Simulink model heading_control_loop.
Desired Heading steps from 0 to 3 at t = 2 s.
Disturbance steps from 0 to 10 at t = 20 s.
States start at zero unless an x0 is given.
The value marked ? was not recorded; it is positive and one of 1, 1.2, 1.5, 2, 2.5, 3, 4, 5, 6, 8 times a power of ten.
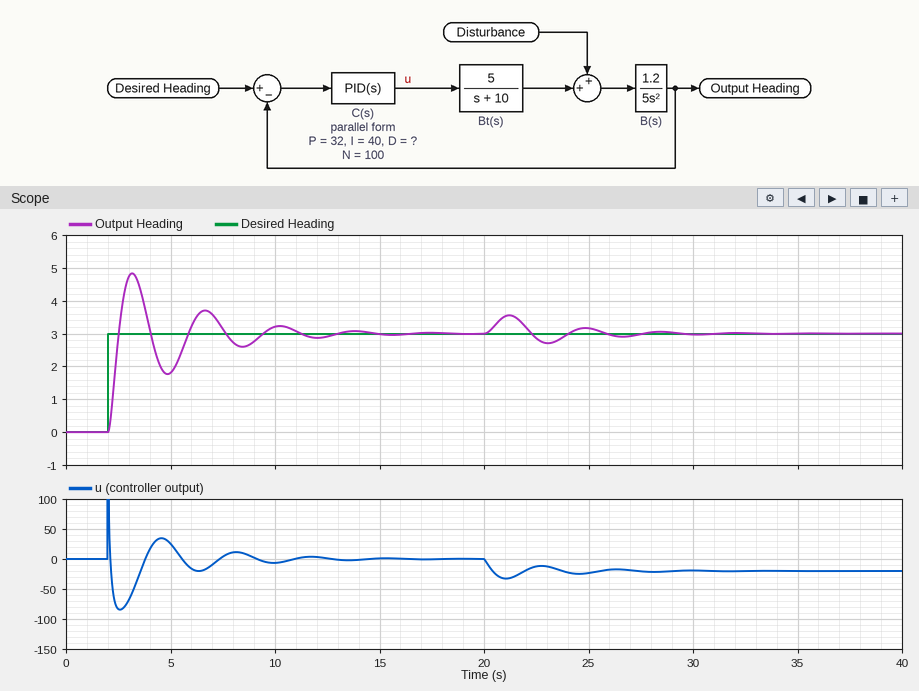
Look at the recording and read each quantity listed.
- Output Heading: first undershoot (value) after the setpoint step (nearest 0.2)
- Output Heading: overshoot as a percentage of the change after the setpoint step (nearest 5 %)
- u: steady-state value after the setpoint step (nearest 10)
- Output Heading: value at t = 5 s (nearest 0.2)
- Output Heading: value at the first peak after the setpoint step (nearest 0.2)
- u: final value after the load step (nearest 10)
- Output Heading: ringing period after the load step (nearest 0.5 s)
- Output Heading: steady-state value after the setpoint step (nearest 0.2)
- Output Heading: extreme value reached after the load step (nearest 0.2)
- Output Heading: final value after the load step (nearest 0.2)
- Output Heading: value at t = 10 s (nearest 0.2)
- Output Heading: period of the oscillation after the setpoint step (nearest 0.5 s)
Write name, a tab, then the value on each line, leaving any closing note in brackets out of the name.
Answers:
Output Heading: first undershoot (value) after the setpoint step	1.8
Output Heading: overshoot as a percentage of the change after the setpoint step	60 %
u: steady-state value after the setpoint step	0
Output Heading: value at t = 5 s	1.8
Output Heading: value at the first peak after the setpoint step	4.8
u: final value after the load step	-20
Output Heading: ringing period after the load step	3.5 s
Output Heading: steady-state value after the setpoint step	3.0
Output Heading: extreme value reached after the load step	3.6
Output Heading: final value after the load step	3.0
Output Heading: value at t = 10 s	3.2
Output Heading: period of the oscillation after the setpoint step	3.5 s
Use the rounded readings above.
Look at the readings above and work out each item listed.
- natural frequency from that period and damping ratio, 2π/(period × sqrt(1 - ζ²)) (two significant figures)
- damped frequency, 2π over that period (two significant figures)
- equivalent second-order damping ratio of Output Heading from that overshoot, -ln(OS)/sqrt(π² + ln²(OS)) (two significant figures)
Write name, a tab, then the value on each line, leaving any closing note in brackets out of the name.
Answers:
natural frequency from that period and damping ratio, 2π/(period × sqrt(1 - ζ²))	1.8 rad/s
damped frequency, 2π over that period	1.8 rad/s
equivalent second-order damping ratio of Output Heading from that overshoot, -ln(OS)/sqrt(π² + ln²(OS))	0.16
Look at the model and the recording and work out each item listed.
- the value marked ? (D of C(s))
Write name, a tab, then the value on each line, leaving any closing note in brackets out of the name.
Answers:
the value marked ? (D of C(s))	20
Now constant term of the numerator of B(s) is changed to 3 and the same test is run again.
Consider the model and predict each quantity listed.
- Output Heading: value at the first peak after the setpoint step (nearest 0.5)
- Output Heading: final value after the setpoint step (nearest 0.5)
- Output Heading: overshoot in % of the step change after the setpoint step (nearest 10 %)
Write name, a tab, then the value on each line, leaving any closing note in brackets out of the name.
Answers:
Output Heading: value at the first peak after the setpoint step	4.5
Output Heading: final value after the setpoint step	3.0
Output Heading: overshoot in % of the step change after the setpoint step	40 %
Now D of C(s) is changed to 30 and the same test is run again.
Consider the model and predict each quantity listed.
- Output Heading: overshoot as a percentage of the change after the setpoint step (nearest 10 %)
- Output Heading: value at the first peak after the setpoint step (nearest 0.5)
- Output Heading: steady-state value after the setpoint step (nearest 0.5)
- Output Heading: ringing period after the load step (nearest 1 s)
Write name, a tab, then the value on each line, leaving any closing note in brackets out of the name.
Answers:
Output Heading: overshoot as a percentage of the change after the setpoint step	40 %
Output Heading: value at the first peak after the setpoint step	4.0
Output Heading: steady-state value after the setpoint step	3.0
Output Heading: ringing period after the load step	5 s
